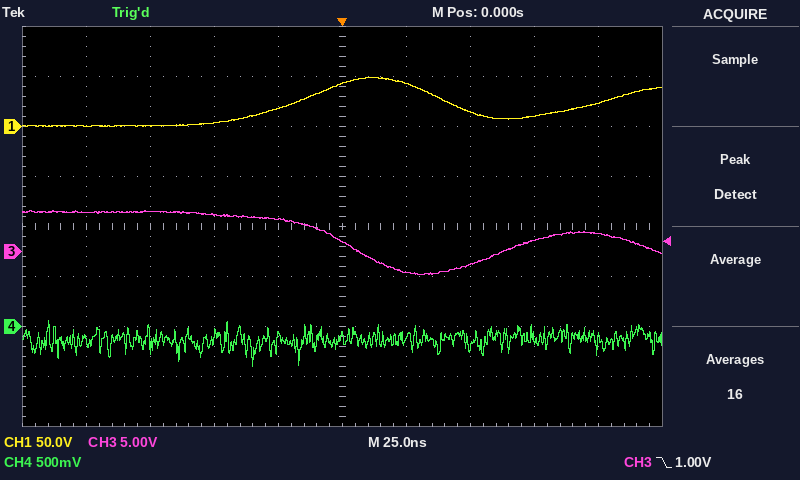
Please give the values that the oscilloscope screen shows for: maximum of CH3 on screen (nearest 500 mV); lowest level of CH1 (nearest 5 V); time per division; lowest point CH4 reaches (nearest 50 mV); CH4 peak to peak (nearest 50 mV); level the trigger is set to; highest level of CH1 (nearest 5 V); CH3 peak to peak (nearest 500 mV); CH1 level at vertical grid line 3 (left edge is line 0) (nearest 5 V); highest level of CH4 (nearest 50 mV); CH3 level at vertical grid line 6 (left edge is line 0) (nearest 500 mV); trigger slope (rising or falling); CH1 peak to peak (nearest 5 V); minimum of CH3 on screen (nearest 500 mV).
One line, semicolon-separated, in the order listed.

4.0 V; 0 V; 25 ns; -400 mV; 450 mV; 1.00 V; 50 V; 6.5 V; 5 V; 50 mV; -2.0 V; falling; 50 V; -2.5 V
